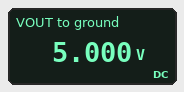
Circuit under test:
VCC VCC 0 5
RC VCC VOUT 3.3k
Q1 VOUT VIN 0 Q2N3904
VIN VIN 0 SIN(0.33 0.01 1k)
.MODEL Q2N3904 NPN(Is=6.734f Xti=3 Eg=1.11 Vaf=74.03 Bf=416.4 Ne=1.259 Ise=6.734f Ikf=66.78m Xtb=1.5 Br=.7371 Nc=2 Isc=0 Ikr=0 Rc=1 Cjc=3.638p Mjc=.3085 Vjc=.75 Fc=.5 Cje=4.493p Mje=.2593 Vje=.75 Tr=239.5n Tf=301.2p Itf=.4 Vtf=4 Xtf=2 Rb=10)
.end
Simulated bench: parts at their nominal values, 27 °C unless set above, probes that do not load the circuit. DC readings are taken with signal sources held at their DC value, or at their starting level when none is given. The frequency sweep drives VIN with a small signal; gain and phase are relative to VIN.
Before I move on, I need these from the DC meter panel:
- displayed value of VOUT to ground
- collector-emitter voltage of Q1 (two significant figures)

5.000 V
5.0 V
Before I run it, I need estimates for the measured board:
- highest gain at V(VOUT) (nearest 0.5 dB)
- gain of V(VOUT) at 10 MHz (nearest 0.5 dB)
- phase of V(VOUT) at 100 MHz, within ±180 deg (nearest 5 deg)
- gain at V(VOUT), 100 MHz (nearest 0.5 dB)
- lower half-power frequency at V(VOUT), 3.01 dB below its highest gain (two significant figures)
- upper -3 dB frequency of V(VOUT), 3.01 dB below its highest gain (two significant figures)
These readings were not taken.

0 dB
-8.5 dB
10 deg
-0.5 dB
24 MHz
3.1 GHz
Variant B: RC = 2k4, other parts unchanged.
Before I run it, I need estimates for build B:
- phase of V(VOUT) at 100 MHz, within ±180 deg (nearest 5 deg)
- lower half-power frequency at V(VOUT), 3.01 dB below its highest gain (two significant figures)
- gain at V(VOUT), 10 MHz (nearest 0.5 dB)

15 deg
33 MHz
-11.0 dB
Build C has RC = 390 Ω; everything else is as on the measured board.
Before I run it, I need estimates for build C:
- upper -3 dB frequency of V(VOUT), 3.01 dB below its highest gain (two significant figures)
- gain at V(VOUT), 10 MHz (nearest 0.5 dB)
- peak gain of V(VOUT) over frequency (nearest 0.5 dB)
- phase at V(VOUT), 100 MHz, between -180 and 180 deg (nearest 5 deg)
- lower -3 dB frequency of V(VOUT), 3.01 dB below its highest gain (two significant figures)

3.5 GHz
-26.5 dB
-1.0 dB
60 deg
180 MHz
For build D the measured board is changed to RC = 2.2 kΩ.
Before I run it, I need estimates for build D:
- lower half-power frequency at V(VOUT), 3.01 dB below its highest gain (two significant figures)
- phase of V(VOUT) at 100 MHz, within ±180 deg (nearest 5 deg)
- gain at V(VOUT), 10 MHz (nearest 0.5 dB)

36 MHz
20 deg
-11.5 dB
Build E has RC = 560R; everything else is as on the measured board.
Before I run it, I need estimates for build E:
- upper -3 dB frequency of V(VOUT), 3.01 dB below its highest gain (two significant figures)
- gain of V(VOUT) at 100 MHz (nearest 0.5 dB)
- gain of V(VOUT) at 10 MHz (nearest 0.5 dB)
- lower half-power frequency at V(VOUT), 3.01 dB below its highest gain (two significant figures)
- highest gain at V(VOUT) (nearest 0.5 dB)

3.4 GHz
-5.0 dB
-23.0 dB
130 MHz
-0.5 dB
